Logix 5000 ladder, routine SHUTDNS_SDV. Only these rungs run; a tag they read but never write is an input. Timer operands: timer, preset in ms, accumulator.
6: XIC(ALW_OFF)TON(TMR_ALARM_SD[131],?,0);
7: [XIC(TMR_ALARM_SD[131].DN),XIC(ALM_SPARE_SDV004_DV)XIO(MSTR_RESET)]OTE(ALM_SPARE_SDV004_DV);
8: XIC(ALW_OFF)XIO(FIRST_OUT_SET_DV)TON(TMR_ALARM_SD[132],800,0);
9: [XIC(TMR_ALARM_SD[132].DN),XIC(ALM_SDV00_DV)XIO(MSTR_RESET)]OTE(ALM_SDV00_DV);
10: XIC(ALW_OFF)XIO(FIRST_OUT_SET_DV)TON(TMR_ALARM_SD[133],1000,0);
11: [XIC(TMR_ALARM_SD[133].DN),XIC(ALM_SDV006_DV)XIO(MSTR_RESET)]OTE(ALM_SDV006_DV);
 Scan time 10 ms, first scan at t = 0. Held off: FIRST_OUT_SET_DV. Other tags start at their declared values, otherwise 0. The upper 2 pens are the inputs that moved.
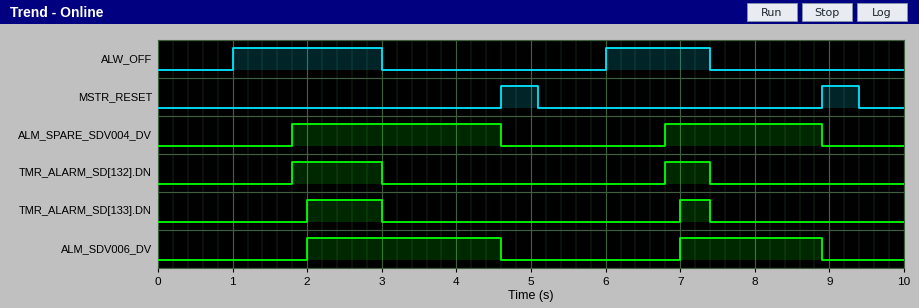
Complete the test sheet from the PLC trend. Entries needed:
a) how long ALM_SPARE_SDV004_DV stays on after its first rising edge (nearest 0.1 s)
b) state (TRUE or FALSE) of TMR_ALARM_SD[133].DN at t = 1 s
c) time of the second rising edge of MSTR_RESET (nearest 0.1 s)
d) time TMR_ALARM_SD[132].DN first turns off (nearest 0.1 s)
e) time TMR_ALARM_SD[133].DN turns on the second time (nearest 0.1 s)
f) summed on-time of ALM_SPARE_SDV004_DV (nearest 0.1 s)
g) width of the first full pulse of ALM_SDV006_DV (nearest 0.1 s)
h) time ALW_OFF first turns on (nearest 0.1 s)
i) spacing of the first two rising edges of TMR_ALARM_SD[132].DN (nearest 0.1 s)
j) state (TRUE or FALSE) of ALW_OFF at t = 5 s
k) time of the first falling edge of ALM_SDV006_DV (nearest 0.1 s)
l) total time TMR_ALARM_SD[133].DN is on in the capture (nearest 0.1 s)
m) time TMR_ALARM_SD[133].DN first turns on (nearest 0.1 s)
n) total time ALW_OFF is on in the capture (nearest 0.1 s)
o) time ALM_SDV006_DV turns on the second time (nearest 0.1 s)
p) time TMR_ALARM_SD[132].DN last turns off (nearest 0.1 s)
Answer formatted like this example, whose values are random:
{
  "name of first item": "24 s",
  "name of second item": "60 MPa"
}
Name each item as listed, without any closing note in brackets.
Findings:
{
  "how long ALM_SPARE_SDV004_DV stays on after its first rising edge": "2.8 s",
  "state (TRUE or FALSE) of TMR_ALARM_SD[133].DN at t = 1 s": "FALSE",
  "time of the second rising edge of MSTR_RESET": "8.9 s",
  "time TMR_ALARM_SD[132].DN first turns off": "3.0 s",
  "time TMR_ALARM_SD[133].DN turns on the second time": "7.0 s",
  "summed on-time of ALM_SPARE_SDV004_DV": "4.9 s",
  "width of the first full pulse of ALM_SDV006_DV": "2.6 s",
  "time ALW_OFF first turns on": "1.0 s",
  "spacing of the first two rising edges of TMR_ALARM_SD[132].DN": "5.0 s",
  "state (TRUE or FALSE) of ALW_OFF at t = 5 s": "FALSE",
  "time of the first falling edge of ALM_SDV006_DV": "4.6 s",
  "total time TMR_ALARM_SD[133].DN is on in the capture": "1.4 s",
  "time TMR_ALARM_SD[133].DN first turns on": "2.0 s",
  "total time ALW_OFF is on in the capture": "3.4 s",
  "time ALM_SDV006_DV turns on the second time": "7.0 s",
  "time TMR_ALARM_SD[132].DN last turns off": "7.4 s"
}
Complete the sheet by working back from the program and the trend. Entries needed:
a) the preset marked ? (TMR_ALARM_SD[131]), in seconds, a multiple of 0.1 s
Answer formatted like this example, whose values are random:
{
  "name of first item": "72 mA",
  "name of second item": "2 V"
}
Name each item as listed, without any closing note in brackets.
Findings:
{
  "the preset marked ? (TMR_ALARM_SD[131]), in seconds, a multiple of 0.1 s": "0.8 s"
}
